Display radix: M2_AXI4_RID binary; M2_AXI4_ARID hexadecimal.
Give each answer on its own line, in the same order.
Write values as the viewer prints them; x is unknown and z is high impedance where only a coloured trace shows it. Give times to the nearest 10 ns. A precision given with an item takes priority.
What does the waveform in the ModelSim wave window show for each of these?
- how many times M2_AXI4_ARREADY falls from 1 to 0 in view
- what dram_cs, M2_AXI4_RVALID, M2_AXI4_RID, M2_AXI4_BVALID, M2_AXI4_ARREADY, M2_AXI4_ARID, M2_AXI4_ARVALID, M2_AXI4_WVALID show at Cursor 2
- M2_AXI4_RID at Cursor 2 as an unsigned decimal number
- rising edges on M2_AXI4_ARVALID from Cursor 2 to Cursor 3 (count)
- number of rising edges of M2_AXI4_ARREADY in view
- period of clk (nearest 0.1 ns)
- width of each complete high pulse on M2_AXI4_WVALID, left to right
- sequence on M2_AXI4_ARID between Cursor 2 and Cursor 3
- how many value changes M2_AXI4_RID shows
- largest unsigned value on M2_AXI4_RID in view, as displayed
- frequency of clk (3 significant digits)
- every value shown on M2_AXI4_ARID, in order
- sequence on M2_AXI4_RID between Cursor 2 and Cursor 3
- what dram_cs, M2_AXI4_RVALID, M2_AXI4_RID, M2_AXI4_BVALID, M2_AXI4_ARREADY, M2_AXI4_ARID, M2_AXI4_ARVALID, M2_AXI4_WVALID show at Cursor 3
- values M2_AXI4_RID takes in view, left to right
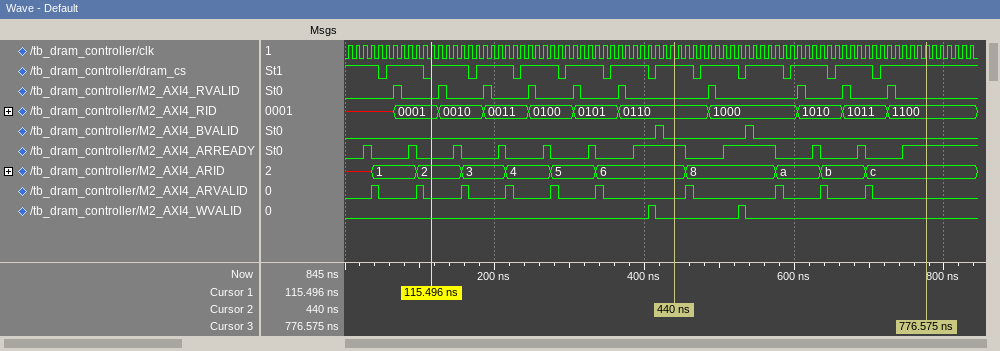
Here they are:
10
dram_cs=1, M2_AXI4_RVALID=0, M2_AXI4_RID=0110, M2_AXI4_BVALID=0, M2_AXI4_ARREADY=1, M2_AXI4_ARID=6, M2_AXI4_ARVALID=0, M2_AXI4_WVALID=0
6
4
11
10 ns
10 ns, 10 ns
6, 8, a, b, c
10
1100
100 MHz
x, 1, 2, 3, 4, 5, 6, 8, a, b, c
0110, 1000, 1010, 1011, 1100
dram_cs=1, M2_AXI4_RVALID=0, M2_AXI4_RID=1100, M2_AXI4_BVALID=0, M2_AXI4_ARREADY=1, M2_AXI4_ARID=c, M2_AXI4_ARVALID=0, M2_AXI4_WVALID=0
x, 0001, 0010, 0011, 0100, 0101, 0110, 1000, 1010, 1011, 1100
